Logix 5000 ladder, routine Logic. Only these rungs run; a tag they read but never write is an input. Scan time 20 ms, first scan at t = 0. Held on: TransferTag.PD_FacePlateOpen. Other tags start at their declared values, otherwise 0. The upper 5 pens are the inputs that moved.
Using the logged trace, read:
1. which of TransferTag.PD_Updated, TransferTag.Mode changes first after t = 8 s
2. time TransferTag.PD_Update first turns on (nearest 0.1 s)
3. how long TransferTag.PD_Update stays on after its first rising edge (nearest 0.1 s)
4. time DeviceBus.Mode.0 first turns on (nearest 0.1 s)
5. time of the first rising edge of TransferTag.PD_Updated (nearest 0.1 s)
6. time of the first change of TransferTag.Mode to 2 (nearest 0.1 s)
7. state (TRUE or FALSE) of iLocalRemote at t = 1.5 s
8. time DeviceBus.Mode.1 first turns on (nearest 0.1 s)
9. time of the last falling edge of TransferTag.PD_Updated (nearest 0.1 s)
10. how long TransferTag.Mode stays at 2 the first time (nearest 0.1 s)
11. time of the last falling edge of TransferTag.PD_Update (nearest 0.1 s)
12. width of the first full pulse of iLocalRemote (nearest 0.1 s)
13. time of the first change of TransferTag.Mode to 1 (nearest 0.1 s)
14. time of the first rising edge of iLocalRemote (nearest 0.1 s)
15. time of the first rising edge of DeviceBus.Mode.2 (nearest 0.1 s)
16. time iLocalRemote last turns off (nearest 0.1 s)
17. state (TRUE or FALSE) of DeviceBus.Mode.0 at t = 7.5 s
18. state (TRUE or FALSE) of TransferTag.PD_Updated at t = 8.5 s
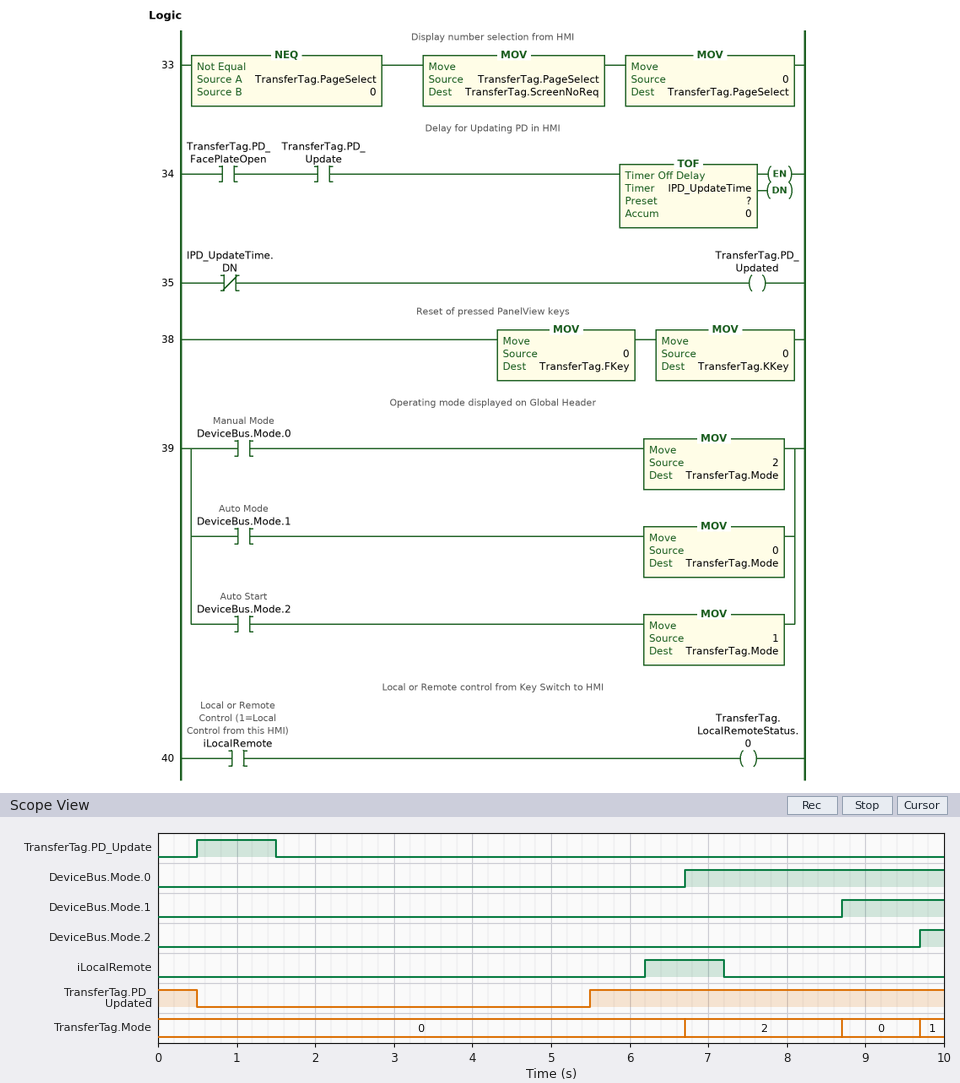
TransferTag.Mode
0.5 s
1.0 s
6.7 s
5.5 s
6.7 s
FALSE
8.7 s
0.5 s
2.0 s
1.5 s
1.0 s
9.7 s
6.2 s
9.7 s
7.2 s
TRUE
TRUE
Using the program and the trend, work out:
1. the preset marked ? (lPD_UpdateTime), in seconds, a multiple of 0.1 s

4.0 s
